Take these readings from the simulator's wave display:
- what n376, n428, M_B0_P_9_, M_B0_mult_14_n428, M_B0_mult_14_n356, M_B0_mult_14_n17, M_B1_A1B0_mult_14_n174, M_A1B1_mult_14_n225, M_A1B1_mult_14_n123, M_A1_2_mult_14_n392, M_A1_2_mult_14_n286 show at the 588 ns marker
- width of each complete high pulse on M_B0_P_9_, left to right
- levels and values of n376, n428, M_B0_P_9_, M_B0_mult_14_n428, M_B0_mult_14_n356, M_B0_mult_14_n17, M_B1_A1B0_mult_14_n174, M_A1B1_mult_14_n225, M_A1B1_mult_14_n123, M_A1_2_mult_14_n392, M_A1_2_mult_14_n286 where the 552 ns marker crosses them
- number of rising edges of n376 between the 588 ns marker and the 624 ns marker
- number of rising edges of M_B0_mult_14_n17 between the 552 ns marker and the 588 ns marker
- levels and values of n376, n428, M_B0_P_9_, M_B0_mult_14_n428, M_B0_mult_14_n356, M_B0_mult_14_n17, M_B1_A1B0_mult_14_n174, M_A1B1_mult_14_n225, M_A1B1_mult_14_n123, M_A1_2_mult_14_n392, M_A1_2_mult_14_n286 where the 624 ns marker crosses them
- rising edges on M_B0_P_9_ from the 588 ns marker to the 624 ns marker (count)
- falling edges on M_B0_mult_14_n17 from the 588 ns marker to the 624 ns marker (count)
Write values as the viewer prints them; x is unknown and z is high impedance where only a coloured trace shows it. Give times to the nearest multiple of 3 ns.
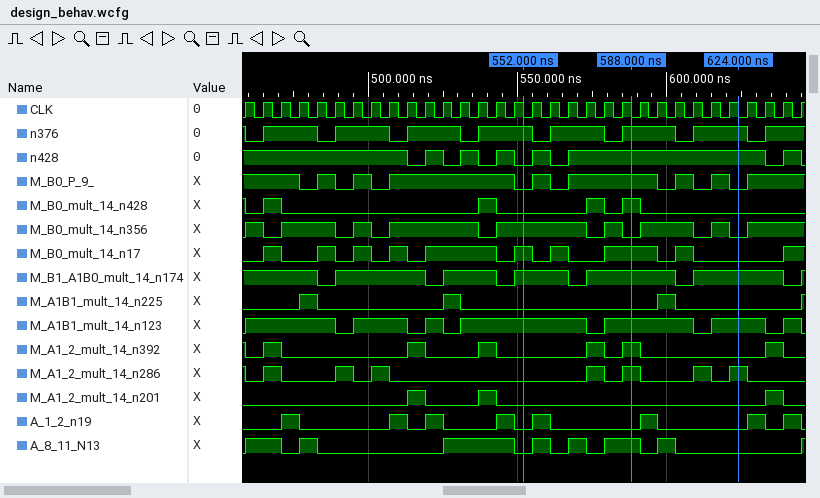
n376=1, n428=1, M_B0_P_9_=1, M_B0_mult_14_n428=1, M_B0_mult_14_n356=0, M_B0_mult_14_n17=1, M_B1_A1B0_mult_14_n174=1, M_A1B1_mult_14_n225=0, M_A1B1_mult_14_n123=1, M_A1_2_mult_14_n392=1, M_A1_2_mult_14_n286=1
6 ns, 6 ns, 42 ns, 6 ns, 30 ns, 6 ns, 6 ns
n376=1, n428=0, M_B0_P_9_=0, M_B0_mult_14_n428=0, M_B0_mult_14_n356=1, M_B0_mult_14_n17=1, M_B1_A1B0_mult_14_n174=1, M_A1B1_mult_14_n225=0, M_A1B1_mult_14_n123=1, M_A1_2_mult_14_n392=0, M_A1_2_mult_14_n286=0
1
2
n376=1, n428=1, M_B0_P_9_=0, M_B0_mult_14_n428=0, M_B0_mult_14_n356=0, M_B0_mult_14_n17=0, M_B1_A1B0_mult_14_n174=1, M_A1B1_mult_14_n225=0, M_A1B1_mult_14_n123=1, M_A1_2_mult_14_n392=0, M_A1_2_mult_14_n286=1
2
2
